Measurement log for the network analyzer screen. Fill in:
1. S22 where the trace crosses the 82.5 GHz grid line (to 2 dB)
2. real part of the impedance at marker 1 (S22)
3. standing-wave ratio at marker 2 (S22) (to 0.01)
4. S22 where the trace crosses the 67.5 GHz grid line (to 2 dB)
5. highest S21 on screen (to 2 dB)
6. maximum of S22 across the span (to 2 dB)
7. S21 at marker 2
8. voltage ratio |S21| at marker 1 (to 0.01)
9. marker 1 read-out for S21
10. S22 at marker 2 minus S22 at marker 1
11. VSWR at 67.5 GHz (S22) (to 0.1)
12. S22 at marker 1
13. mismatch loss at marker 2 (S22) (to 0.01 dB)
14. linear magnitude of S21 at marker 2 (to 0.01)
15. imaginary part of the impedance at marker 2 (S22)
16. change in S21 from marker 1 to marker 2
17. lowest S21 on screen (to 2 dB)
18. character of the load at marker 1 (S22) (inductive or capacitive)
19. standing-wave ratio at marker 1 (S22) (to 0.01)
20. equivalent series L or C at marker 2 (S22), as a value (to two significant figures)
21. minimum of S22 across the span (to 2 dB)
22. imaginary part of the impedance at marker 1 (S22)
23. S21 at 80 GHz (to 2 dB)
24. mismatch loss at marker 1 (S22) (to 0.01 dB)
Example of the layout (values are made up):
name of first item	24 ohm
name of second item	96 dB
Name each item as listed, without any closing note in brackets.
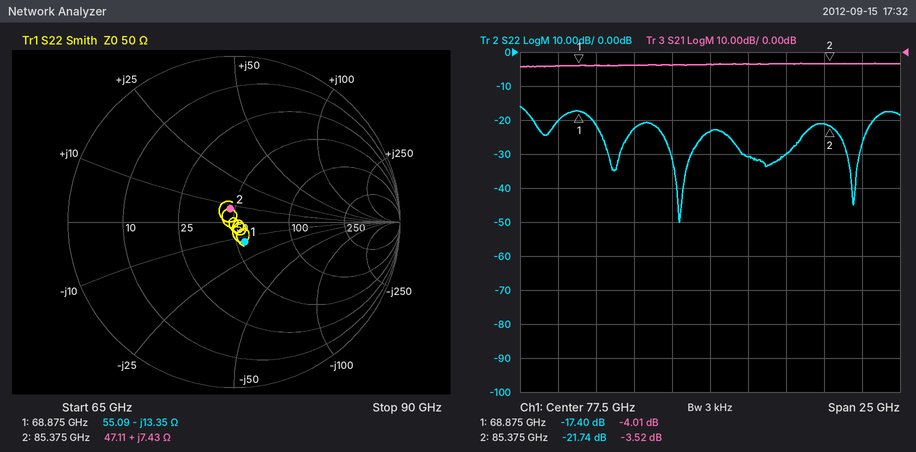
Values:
S22 where the trace crosses the 82.5 GHz grid line	-30 dB
real part of the impedance at marker 1	55.09 Ω
standing-wave ratio at marker 2 (S22)	1.18
S22 where the trace crosses the 67.5 GHz grid line	-20 dB
highest S21 on screen	-4 dB
maximum of S22 across the span	-16 dB
S21 at marker 2	-3.52 dB
voltage ratio |S21| at marker 1	0.63
marker 1 read-out for S21	-4.01 dB
S22 at marker 2 minus S22 at marker 1	-4.34 dB
VSWR at 67.5 GHz (S22)	1.2
S22 at marker 1	-17.40 dB
mismatch loss at marker 2 (S22)	0.03 dB
linear magnitude of S21 at marker 2	0.67
imaginary part of the impedance at marker 2	+7.43 Ω
change in S21 from marker 1 to marker 2	0.49 dB
lowest S21 on screen	-4 dB
character of the load at marker 1 (S22)	capacitive
standing-wave ratio at marker 1 (S22)	1.31
equivalent series L or C at marker 2 (S22), as a value	14 pH
minimum of S22 across the span	-50 dB
imaginary part of the impedance at marker 1	-13.35 Ω
S21 at 80 GHz	-4 dB
mismatch loss at marker 1 (S22)	0.08 dB
